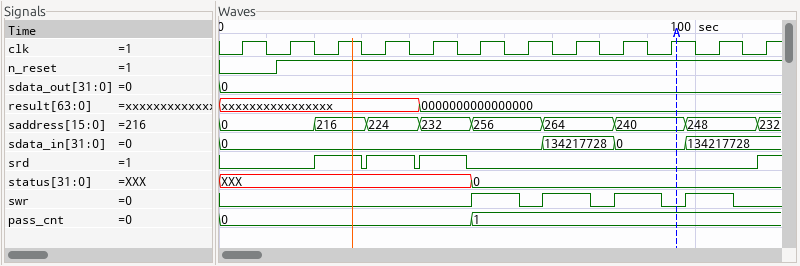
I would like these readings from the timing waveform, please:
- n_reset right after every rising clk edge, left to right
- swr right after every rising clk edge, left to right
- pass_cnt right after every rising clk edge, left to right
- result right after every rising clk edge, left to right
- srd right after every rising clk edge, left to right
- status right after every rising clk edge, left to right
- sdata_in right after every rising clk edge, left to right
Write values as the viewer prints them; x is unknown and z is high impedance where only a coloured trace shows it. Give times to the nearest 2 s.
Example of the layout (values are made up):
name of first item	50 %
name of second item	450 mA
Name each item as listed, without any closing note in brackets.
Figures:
n_reset right after every rising clk edge, left to right	0 1 1 1 1 1 1 1 1 1 1 1
swr right after every rising clk edge, left to right	0 0 0 0 0 1 0 1 1 0 1 0
pass_cnt right after every rising clk edge, left to right	0, 0, 0, 0, 0, 1, 1, 1, 1, 1, 1, 1
result right after every rising clk edge, left to right	xxxxxxxxxxxxxxxx, xxxxxxxxxxxxxxxx, xxxxxxxxxxxxxxxx, xxxxxxxxxxxxxxxx, 0000000000000000, 0000000000000000, 0000000000000000, 0000000000000000, 0000000000000000, 0000000000000000, 0000000000000000, 0000000000000000
srd right after every rising clk edge, left to right	0 0 1 1 1 0 0 0 0 0 0 1
status right after every rising clk edge, left to right	XXX, XXX, XXX, XXX, XXX, 0, 0, 0, 0, 0, 0, 0
sdata_in right after every rising clk edge, left to right	0, 0, 0, 0, 0, 0, 0, 134217728, 0, 0, 134217728, 134217728
